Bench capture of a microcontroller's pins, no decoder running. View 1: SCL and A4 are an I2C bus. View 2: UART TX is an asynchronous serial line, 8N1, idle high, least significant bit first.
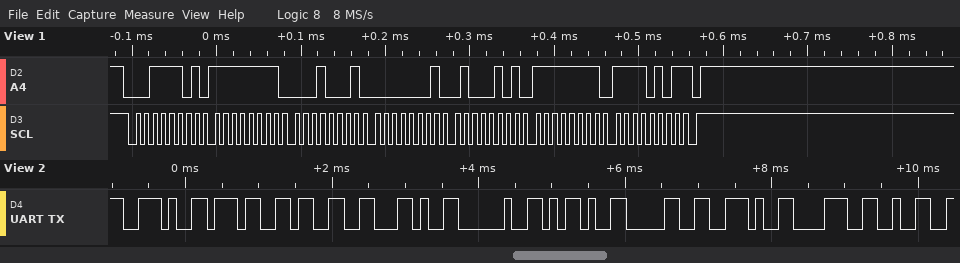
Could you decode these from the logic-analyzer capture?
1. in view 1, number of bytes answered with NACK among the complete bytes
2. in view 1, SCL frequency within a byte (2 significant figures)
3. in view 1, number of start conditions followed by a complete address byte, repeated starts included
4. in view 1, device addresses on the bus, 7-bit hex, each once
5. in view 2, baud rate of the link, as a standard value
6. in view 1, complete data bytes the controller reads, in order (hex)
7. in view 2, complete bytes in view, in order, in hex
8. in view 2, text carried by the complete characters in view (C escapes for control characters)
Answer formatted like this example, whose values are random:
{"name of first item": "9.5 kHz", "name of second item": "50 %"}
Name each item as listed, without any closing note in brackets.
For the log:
{"in view 1, number of bytes answered with NACK among the complete bytes": "1", "in view 1, SCL frequency within a byte": "100 kHz", "in view 1, number of start conditions followed by a complete address byte, repeated starts included": "1", "in view 1, device addresses on the bus, 7-bit hex, each once": "0x1E", "in view 2, baud rate of the link, as a standard value": "9600 baud", "in view 1, complete data bytes the controller reads, in order": "FF 11 01 45 FF F5", "in view 2, complete bytes in view, in order, in hex": "2E 37 33 2C 20 2D 30 2E 38 32", "in view 2, text carried by the complete characters in view": "\".73, -0.82\""}
